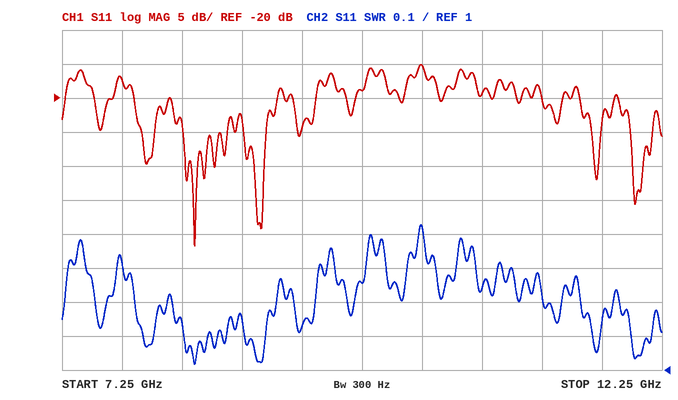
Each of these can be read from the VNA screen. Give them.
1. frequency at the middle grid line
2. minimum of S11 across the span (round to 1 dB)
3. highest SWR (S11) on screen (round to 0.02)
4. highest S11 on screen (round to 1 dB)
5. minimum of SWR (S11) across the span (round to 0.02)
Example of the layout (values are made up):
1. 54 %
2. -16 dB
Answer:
1. 9.75 GHz
2. -42 dB
3. 1.42
4. -15 dB
5. 1.02
